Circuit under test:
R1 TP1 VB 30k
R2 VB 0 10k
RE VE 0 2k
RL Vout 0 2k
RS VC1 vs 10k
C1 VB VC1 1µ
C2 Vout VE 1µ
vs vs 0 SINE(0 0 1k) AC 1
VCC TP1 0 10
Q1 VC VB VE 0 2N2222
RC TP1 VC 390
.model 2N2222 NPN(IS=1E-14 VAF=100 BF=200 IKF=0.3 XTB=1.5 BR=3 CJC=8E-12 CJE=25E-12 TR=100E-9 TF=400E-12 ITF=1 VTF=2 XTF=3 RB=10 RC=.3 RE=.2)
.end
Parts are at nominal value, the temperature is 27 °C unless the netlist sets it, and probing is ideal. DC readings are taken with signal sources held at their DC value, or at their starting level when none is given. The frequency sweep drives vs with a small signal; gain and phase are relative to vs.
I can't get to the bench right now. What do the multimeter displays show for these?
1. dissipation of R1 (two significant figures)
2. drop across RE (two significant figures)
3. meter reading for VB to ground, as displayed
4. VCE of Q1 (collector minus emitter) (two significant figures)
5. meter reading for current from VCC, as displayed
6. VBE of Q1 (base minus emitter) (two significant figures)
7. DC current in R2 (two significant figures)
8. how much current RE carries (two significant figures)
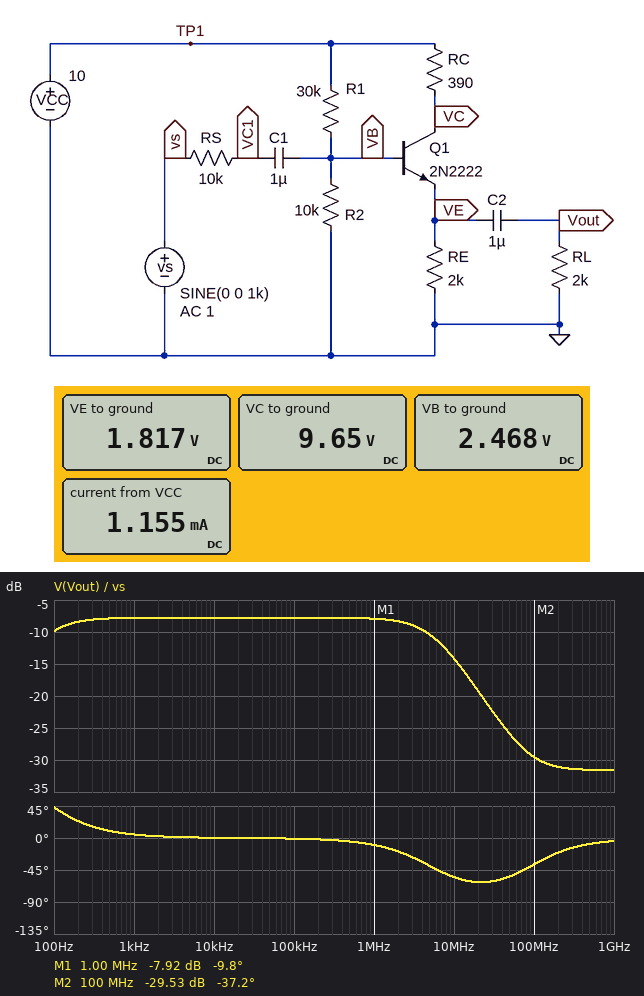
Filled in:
1.9 mW
1.8 V
2.468 V
7.8 V
1.155 mA
650 mV
250 µA
910 µA
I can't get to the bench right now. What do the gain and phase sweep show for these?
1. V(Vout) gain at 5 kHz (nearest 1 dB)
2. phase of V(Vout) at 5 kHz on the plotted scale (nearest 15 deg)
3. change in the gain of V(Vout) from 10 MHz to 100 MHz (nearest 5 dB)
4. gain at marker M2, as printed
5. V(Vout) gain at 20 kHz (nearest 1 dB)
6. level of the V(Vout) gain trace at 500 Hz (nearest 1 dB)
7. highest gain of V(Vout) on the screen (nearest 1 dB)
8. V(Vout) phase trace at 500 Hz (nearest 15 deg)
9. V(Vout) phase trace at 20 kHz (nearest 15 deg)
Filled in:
-8 dB
0 deg
-15 dB
-29.53 dB
-8 dB
-8 dB
-8 dB
15 deg
0 deg
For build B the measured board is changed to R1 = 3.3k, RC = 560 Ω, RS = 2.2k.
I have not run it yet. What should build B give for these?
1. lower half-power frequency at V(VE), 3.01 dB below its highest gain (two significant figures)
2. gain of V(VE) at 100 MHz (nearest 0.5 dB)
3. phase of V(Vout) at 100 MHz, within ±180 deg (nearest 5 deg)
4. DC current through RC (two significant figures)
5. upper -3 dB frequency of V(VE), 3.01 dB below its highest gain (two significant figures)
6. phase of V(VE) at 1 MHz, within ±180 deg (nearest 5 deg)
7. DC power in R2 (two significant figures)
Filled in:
34 Hz
-18.0 dB
-15 deg
3.4 mA
10 MHz
-5 deg
5.6 mW
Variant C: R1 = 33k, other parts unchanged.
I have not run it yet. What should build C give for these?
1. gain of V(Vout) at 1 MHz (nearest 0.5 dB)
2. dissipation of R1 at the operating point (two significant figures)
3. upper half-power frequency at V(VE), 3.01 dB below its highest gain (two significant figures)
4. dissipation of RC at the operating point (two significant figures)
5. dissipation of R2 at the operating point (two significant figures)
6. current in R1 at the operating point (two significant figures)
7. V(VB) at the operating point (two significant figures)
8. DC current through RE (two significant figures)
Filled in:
-8.0 dB
1.8 mW
5.3 MHz
260 µW
530 µW
230 µA
2.3 V
820 µA
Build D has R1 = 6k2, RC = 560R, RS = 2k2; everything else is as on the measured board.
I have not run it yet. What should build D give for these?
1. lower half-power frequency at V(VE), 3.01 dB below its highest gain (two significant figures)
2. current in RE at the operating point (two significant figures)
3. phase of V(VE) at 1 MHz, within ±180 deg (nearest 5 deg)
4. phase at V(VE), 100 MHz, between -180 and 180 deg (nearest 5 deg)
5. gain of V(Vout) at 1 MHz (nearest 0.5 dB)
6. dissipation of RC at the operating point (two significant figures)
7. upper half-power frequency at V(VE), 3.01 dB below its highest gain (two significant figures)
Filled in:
26 Hz
2.7 mA
-5 deg
-20 deg
-4.0 dB
4.1 mW
11 MHz
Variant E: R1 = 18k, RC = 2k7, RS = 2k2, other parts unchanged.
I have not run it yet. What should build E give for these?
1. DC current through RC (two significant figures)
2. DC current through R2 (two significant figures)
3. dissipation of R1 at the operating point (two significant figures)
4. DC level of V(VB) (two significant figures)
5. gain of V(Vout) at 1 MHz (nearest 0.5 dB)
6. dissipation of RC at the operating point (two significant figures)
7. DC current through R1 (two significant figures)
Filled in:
1.4 mA
350 µA
2.3 mW
3.5 V
-3.0 dB
5.5 mW
360 µA
